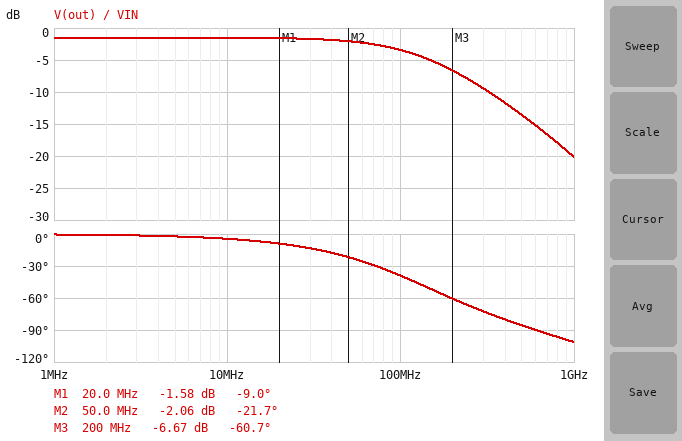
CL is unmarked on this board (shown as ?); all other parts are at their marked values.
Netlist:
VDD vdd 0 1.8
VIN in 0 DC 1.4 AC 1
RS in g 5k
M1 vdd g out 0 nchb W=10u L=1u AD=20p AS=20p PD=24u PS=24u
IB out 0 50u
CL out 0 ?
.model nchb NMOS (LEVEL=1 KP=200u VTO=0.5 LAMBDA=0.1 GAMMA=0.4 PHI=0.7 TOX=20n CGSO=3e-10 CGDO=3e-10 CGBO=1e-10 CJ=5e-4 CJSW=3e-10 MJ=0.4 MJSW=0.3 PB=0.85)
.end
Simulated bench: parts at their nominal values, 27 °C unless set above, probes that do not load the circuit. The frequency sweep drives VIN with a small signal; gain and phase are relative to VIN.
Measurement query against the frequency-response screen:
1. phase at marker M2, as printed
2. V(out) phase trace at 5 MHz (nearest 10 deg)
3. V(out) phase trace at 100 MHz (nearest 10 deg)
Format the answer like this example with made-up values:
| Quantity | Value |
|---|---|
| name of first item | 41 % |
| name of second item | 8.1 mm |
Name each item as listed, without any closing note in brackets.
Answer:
| Quantity | Value |
|---|---|
| phase at marker M2, as printed | -21.7 deg |
| V(out) phase trace at 5 MHz | 0 deg |
| V(out) phase trace at 100 MHz | -40 deg |
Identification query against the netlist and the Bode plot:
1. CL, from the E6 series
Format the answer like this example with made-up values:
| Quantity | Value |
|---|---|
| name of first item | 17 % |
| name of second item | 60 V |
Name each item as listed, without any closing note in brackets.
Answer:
| Quantity | Value |
|---|---|
| CL, from the E6 series | 680 fF |
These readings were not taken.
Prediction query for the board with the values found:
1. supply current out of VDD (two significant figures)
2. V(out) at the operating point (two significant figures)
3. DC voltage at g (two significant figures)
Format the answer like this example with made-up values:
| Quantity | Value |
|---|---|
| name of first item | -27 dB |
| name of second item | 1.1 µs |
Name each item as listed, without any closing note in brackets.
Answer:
| Quantity | Value |
|---|---|
| supply current out of VDD | 50 µA |
| V(out) at the operating point | 570 mV |
| DC voltage at g | 1.4 V |
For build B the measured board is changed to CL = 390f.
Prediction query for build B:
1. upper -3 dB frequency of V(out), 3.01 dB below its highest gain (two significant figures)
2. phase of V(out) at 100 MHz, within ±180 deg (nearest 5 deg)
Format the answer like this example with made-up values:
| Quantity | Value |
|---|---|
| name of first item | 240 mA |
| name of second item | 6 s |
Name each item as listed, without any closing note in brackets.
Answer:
| Quantity | Value |
|---|---|
| upper -3 dB frequency of V(out), 3.01 dB below its highest gain | 230 MHz |
| phase of V(out) at 100 MHz, within ±180 deg | -25 deg |
